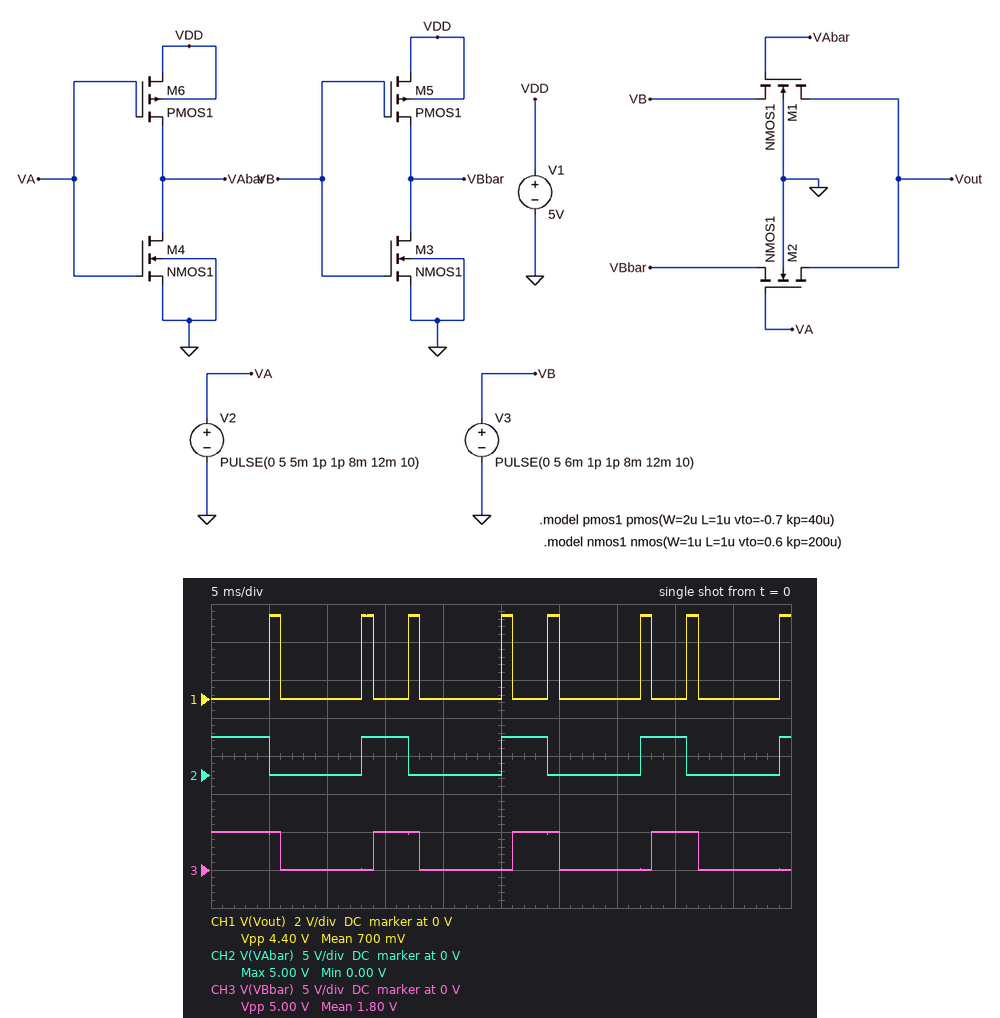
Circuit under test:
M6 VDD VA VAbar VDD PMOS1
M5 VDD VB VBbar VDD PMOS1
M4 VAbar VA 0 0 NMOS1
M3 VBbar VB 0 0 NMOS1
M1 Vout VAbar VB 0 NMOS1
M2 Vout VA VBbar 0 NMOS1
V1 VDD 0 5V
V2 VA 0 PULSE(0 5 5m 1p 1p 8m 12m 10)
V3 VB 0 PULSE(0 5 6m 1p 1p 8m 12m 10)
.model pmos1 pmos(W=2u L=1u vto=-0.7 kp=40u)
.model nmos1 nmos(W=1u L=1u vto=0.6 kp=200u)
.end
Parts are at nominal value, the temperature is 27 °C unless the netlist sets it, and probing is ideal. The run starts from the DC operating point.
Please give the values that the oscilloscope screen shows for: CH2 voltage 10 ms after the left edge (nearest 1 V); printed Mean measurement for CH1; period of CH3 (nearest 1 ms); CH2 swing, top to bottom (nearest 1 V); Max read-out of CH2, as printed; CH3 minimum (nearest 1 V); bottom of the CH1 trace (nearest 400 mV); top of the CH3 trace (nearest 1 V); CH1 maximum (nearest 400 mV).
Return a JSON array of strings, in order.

["0 V", "700 mV", "12 ms", "5 V", "5.00 V", "0 V", "0 V", "5 V", "4.4 V"]
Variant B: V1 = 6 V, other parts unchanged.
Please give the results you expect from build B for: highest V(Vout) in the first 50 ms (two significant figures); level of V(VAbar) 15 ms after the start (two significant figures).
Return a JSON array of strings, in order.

["5.0 V", "6.0 V"]
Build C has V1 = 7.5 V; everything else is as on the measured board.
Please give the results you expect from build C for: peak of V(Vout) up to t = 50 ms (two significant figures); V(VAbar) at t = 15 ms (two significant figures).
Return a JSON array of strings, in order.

["5.0 V", "7.5 V"]
